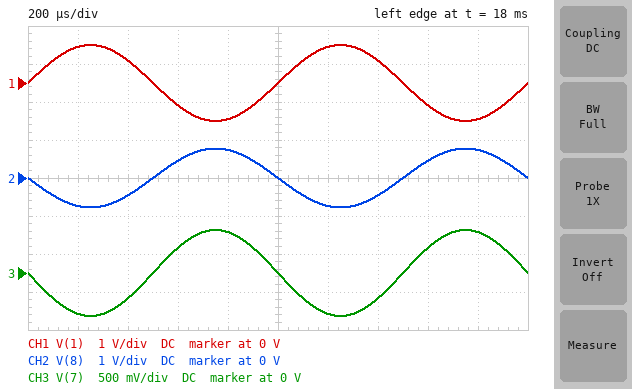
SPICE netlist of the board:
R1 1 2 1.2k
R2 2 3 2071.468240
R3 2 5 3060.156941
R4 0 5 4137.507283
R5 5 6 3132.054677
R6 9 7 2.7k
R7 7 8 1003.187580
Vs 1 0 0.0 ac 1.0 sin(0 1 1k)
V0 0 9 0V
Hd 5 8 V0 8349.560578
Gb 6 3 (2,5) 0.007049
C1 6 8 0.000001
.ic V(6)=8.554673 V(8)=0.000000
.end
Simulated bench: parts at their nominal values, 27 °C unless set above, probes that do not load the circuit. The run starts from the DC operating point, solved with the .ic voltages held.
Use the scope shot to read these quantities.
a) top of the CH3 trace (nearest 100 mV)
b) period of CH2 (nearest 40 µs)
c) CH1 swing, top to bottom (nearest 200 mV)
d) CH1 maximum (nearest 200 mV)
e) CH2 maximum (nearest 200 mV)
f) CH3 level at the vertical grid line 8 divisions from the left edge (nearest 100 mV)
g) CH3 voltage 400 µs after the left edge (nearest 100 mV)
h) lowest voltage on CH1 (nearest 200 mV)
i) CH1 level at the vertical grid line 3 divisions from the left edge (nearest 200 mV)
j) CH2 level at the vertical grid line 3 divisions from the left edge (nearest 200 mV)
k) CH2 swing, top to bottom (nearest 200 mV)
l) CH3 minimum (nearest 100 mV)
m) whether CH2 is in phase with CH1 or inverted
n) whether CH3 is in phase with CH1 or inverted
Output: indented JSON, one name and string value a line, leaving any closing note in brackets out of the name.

{
  "top of the CH3 trace": "600 mV",
  "period of CH2": "1.00 ms",
  "CH1 swing, top to bottom": "2.0 V",
  "CH1 maximum": "1.0 V",
  "CH2 maximum": "800 mV",
  "CH3 level at the vertical grid line 8 divisions from the left edge": "300 mV",
  "CH3 voltage 400 µs after the left edge": "-300 mV",
  "lowest voltage on CH1": "-1.0 V",
  "CH1 level at the vertical grid line 3 divisions from the left edge": "-600 mV",
  "CH2 level at the vertical grid line 3 divisions from the left edge": "400 mV",
  "CH2 swing, top to bottom": "1.6 V",
  "CH3 minimum": "-600 mV",
  "whether CH2 is in phase with CH1 or inverted": "inverted",
  "whether CH3 is in phase with CH1 or inverted": "inverted"
}
